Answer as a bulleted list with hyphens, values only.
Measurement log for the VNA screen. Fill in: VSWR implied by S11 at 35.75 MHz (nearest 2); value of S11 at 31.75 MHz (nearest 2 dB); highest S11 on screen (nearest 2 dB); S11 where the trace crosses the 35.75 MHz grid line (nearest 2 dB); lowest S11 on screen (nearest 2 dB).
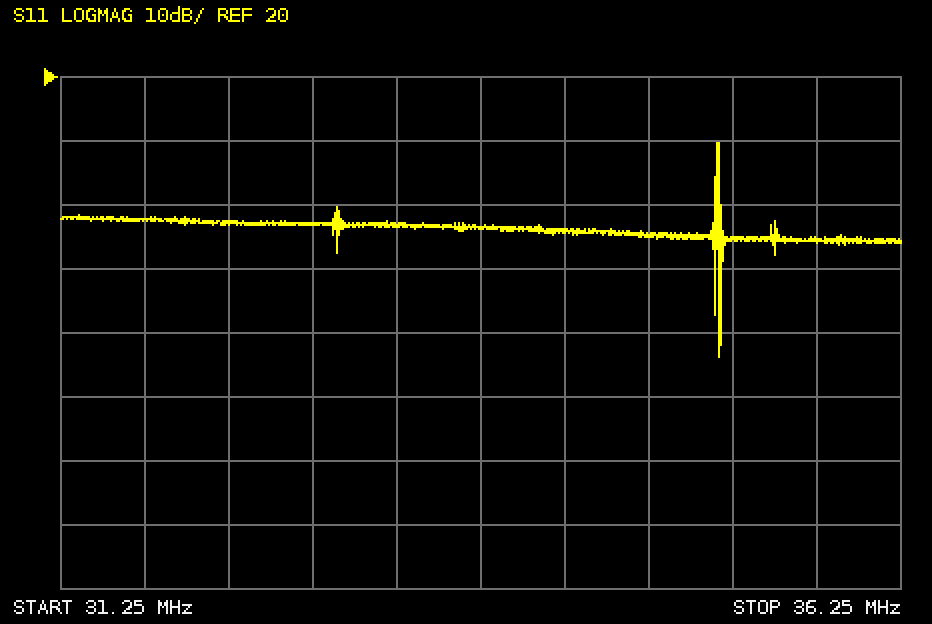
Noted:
- 4
- -2 dB
- 10 dB
- -6 dB
- -24 dB
